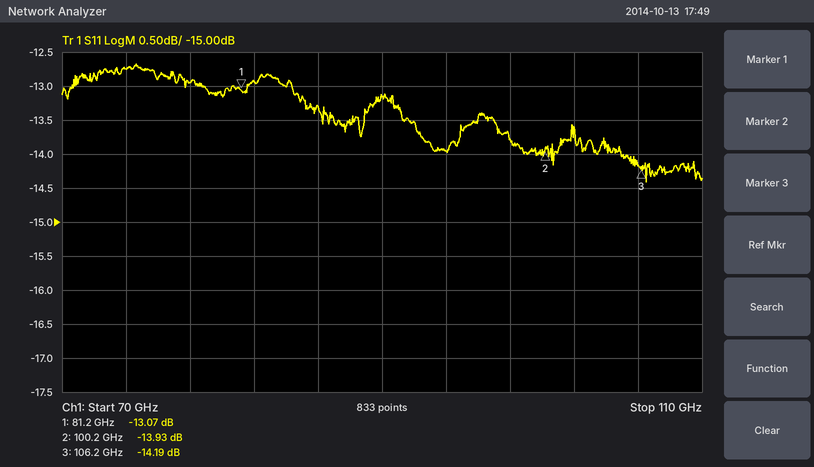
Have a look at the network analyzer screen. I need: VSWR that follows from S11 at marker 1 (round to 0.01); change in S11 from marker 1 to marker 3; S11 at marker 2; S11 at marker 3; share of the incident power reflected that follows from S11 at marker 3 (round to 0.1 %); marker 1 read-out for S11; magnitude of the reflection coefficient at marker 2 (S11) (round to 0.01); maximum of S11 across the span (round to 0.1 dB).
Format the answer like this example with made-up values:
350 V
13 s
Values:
1.57
-1.12 dB
-13.93 dB
-14.19 dB
3.8 %
-13.07 dB
0.20
-12.7 dB
